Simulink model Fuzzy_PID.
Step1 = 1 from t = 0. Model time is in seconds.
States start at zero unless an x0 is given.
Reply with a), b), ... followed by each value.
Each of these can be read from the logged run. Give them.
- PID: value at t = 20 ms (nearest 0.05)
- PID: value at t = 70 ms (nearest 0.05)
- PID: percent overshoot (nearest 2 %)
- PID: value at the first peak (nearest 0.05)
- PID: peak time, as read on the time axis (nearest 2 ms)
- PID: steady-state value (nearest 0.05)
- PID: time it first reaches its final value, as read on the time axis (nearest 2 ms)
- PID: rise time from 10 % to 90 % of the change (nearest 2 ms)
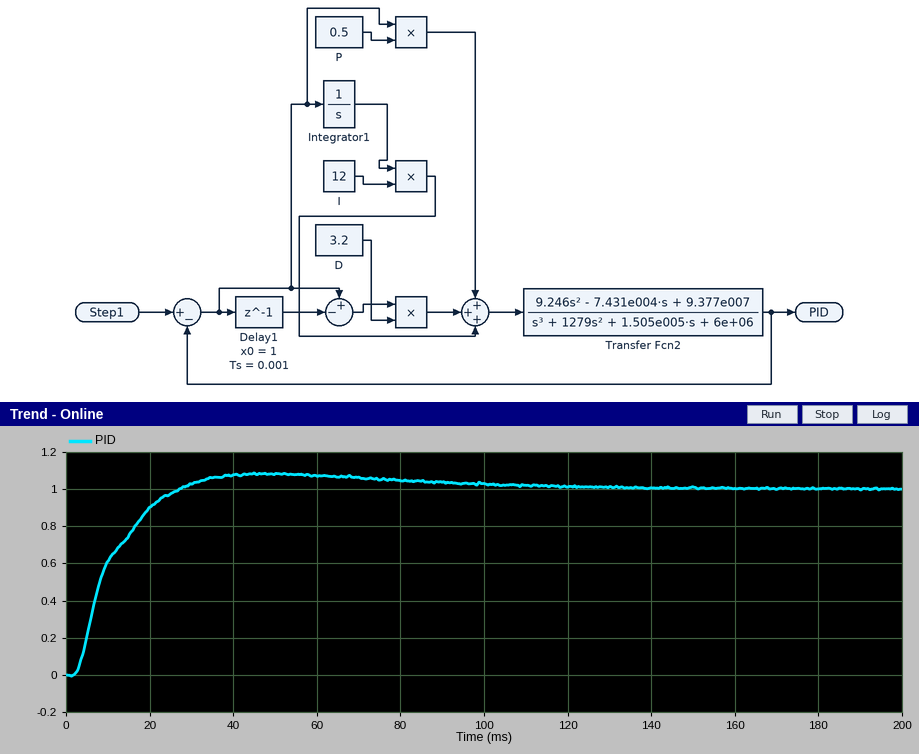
a) 0.90
b) 1.05
c) 8 %
d) 1.10
e) 48 ms
f) 1.00
g) 28 ms
h) 16 ms
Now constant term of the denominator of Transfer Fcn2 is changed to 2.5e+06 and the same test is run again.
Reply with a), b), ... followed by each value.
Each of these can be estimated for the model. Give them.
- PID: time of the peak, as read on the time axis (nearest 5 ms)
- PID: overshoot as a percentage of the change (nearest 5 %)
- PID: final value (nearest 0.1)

a) 45 ms
b) 15 %
c) 1.0
